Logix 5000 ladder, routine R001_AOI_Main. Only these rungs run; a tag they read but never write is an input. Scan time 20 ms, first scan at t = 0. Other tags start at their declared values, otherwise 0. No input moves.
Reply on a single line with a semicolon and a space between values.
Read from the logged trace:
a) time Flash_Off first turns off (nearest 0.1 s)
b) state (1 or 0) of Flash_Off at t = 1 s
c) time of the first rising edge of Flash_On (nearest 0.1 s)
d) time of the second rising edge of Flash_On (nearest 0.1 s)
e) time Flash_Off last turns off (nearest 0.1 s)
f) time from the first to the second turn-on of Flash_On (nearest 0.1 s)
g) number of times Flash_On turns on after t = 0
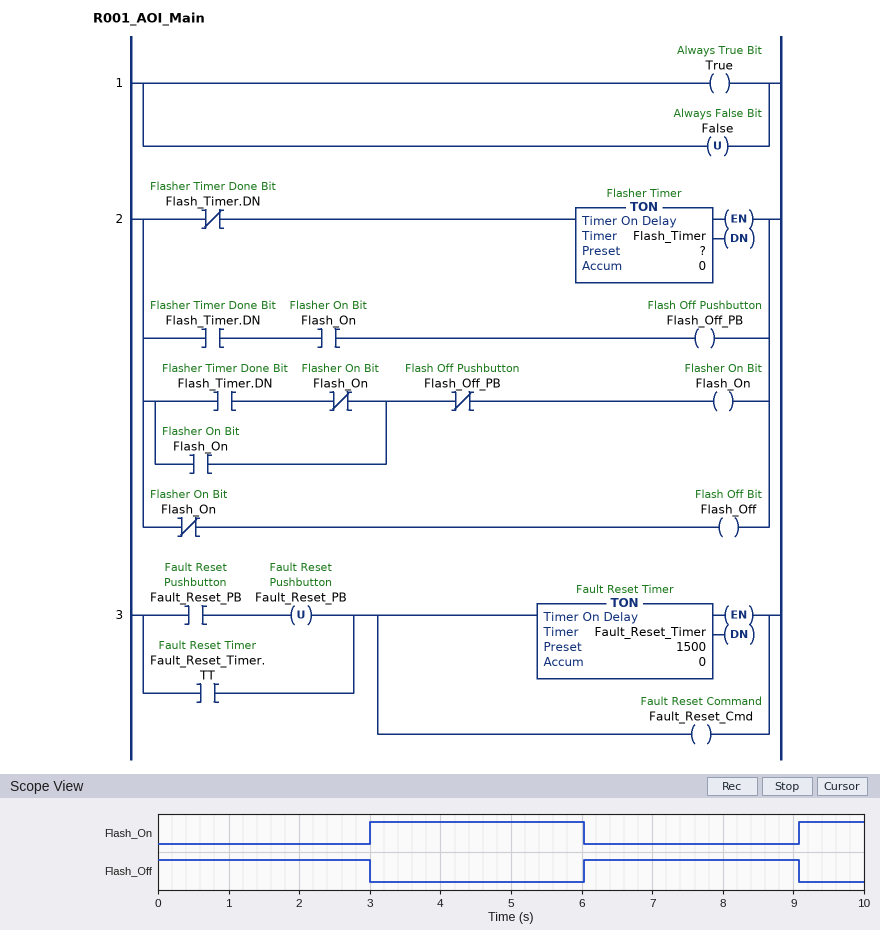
3.0 s; 1; 3.0 s; 9.1 s; 9.1 s; 6.1 s; 2
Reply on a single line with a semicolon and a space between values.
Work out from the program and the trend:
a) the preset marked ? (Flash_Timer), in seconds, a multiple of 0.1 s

3.0 s
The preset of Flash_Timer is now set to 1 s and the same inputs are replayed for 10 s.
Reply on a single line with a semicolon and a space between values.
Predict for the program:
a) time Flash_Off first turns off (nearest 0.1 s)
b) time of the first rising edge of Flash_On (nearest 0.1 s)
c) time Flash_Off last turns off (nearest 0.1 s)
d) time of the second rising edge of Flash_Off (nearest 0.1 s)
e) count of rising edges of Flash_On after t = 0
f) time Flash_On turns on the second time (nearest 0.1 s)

1.0 s; 1.0 s; 9.3 s; 4.1 s; 5; 3.1 s
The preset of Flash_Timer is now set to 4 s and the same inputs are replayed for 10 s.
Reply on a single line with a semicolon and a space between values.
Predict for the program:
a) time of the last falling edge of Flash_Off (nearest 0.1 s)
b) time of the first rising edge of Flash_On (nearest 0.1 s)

4.0 s; 4.0 s
